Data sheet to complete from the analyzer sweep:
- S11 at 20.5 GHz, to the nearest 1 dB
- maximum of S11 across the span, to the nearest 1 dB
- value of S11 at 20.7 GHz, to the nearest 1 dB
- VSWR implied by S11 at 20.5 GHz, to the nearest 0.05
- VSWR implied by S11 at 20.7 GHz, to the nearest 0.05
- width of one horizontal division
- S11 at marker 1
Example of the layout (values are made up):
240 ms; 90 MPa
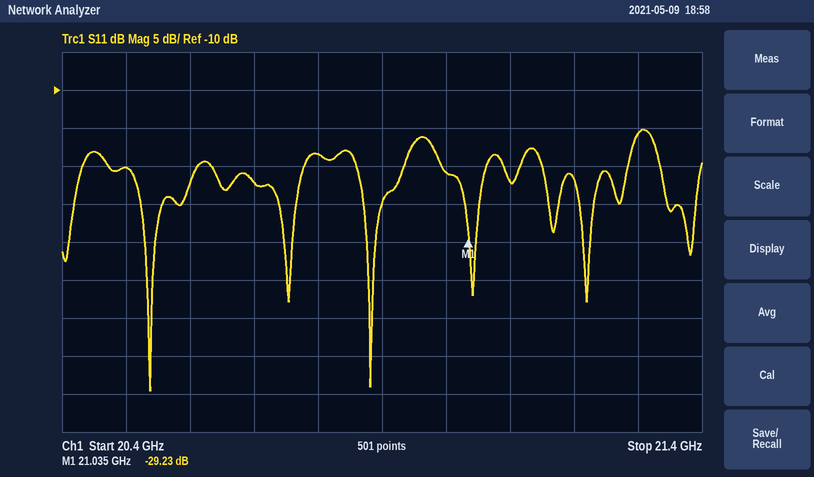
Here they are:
-20 dB; -15 dB; -22 dB; 1.20; 1.15; 100 MHz; -29.23 dB
